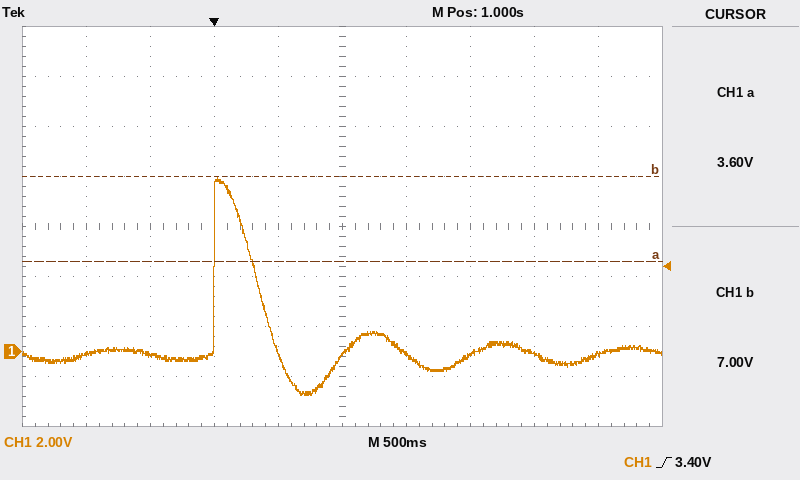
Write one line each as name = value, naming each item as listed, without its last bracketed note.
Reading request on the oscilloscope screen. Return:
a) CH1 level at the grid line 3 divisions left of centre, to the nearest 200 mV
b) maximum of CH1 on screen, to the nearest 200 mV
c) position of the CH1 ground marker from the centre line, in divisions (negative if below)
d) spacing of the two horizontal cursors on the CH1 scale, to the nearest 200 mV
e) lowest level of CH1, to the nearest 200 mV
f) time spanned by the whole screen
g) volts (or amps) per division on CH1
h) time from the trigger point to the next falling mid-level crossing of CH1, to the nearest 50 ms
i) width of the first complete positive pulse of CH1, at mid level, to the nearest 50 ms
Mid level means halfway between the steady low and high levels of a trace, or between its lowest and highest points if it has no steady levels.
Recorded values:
CH1 level at the grid line 3 divisions left of centre, to the nearest 200 mV = -200 mV
maximum of CH1 on screen, to the nearest 200 mV = 7.0 V
position of the CH1 ground marker from the centre line, in divisions = -2.5 div
spacing of the two horizontal cursors on the CH1 scale, to the nearest 200 mV = 3.4 V
lowest level of CH1, to the nearest 200 mV = -1.8 V
time spanned by the whole screen = 5 s
volts (or amps) per division on CH1 = 2 V
time from the trigger point to the next falling mid-level crossing of CH1, to the nearest 50 ms = 350 ms
width of the first complete positive pulse of CH1, at mid level, to the nearest 50 ms = 350 ms
